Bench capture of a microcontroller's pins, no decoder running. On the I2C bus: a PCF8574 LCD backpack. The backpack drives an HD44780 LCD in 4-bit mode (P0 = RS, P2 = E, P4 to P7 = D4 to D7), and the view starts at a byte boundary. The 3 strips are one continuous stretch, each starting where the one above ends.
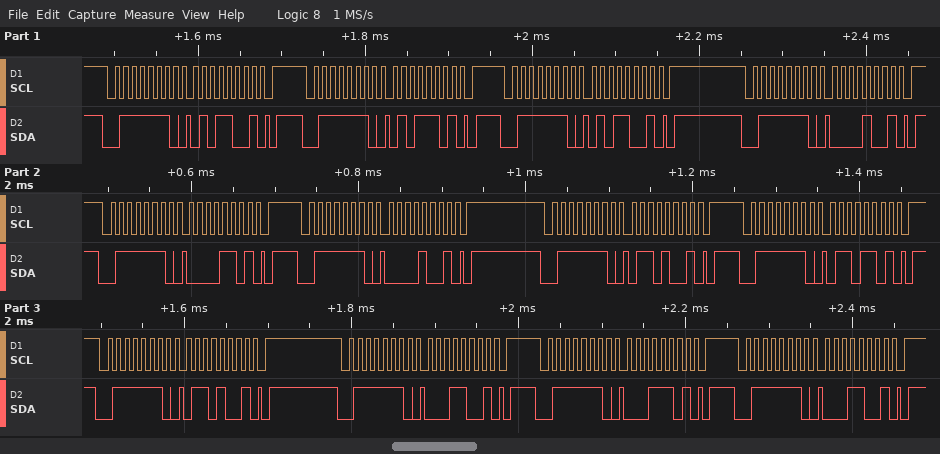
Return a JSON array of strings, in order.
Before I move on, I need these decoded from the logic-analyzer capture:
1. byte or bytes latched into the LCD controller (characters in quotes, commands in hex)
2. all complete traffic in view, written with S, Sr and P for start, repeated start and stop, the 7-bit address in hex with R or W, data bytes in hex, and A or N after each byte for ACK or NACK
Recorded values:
["'P' 'a'", "S 3FW A 59 A P S 3FW A 5D A P S 3FW A 59 A P S 3FW A 09 A P S 3FW A 0D A P S 3FW A 09 A P S 3FW A 69 A P S 3FW A 6D A P S 3FW A 69 A P S 3FW A 19 A P S 3FW A 1D A P S 3FW A 19 A P"]
